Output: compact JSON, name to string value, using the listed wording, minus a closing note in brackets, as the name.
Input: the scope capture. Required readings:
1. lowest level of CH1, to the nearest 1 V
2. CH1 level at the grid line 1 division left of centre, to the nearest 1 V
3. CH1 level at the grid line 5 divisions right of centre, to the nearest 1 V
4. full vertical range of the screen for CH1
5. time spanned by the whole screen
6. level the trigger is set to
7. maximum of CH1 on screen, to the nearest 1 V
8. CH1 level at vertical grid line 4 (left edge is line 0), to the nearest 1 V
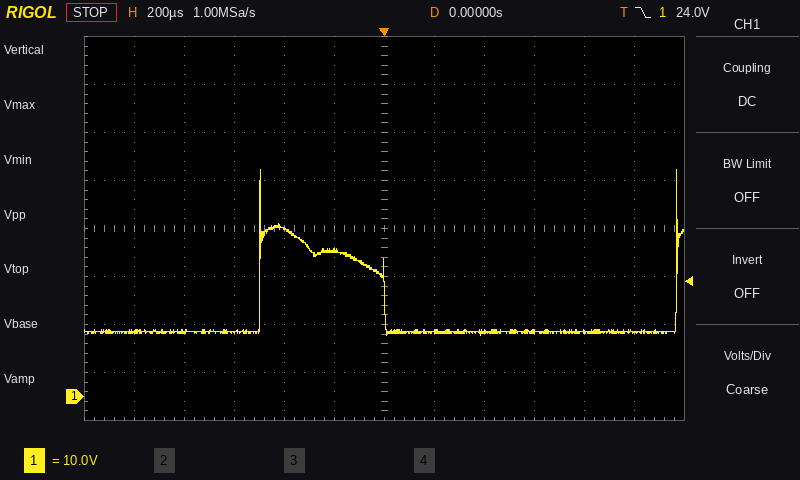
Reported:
{"lowest level of CH1, to the nearest 1 V": "13 V", "CH1 level at the grid line 1 division left of centre, to the nearest 1 V": "30 V", "CH1 level at the grid line 5 divisions right of centre, to the nearest 1 V": "13 V", "full vertical range of the screen for CH1": "80 V", "time spanned by the whole screen": "2.4 ms", "level the trigger is set to": "24.0 V", "maximum of CH1 on screen, to the nearest 1 V": "47 V", "CH1 level at vertical grid line 4 (left edge is line 0), to the nearest 1 V": "35 V"}
